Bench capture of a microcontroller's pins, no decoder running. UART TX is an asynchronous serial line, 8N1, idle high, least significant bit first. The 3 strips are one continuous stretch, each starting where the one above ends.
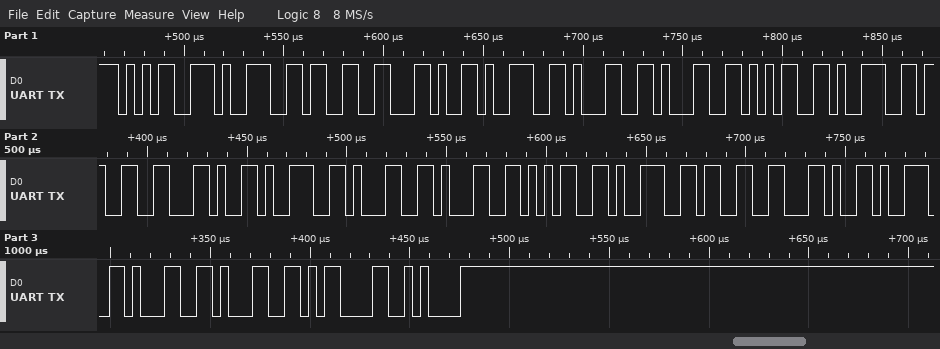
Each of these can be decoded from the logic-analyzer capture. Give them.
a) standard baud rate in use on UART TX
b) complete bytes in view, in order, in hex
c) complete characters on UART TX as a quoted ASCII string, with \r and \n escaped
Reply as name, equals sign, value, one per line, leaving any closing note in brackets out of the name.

standard baud rate in use on UART TX = 250000 baud
complete bytes in view, in order, in hex = 35 39 33 2C 39 31 31 35 39 33 2C 39 31 31 35 39 33 2C 39 31 31 0D 0A
complete characters on UART TX as a quoted ASCII string, with \r and \n escaped = "593,911593,911593,911\r\n"
